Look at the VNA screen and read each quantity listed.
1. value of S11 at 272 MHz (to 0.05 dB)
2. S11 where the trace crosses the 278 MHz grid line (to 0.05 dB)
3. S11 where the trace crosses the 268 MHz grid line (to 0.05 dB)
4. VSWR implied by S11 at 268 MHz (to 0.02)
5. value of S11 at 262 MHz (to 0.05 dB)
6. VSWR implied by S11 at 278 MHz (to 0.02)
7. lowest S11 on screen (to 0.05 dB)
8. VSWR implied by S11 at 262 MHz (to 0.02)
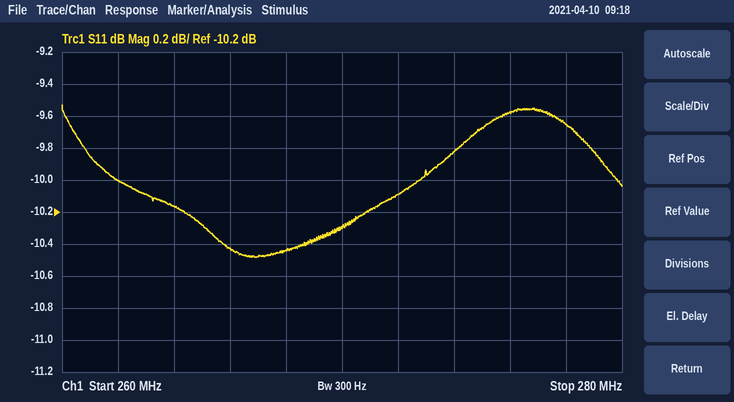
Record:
-10.10 dB
-9.65 dB
-10.45 dB
1.86
-10.00 dB
1.98
-10.50 dB
1.92
